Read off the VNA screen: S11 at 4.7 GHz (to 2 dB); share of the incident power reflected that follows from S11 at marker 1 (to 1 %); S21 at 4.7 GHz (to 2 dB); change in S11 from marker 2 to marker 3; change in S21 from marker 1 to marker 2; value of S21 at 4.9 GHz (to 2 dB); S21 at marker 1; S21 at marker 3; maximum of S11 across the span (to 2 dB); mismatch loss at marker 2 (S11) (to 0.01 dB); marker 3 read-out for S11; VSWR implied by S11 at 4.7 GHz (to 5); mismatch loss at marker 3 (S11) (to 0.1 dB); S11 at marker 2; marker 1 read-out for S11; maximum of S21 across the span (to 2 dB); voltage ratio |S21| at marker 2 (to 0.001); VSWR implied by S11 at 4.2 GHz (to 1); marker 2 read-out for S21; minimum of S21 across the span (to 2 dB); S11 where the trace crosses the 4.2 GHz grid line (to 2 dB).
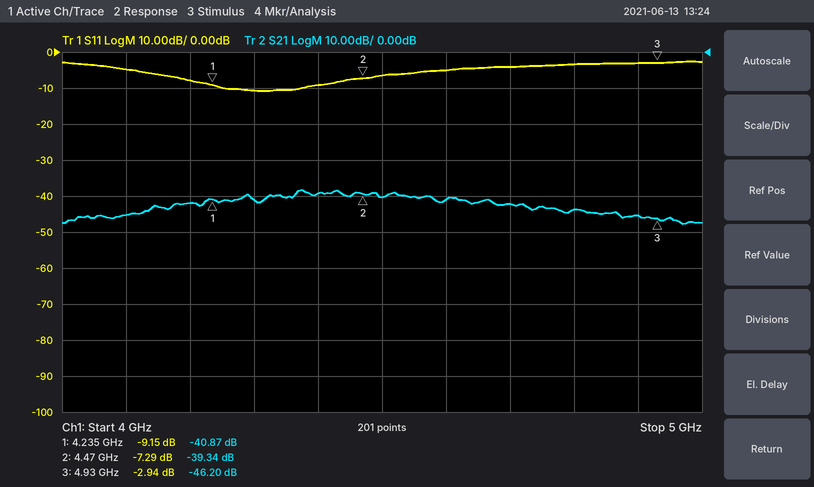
-4 dB
12 %
-42 dB
4.35 dB
1.53 dB
-46 dB
-40.87 dB
-46.20 dB
-2 dB
0.90 dB
-2.94 dB
5
3.1 dB
-7.29 dB
-9.15 dB
-38 dB
0.011
2
-39.34 dB
-48 dB
-8 dB
